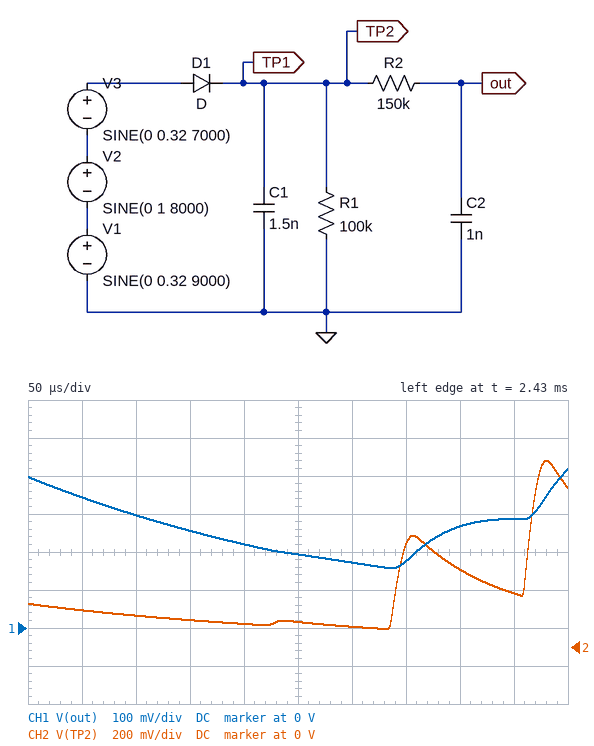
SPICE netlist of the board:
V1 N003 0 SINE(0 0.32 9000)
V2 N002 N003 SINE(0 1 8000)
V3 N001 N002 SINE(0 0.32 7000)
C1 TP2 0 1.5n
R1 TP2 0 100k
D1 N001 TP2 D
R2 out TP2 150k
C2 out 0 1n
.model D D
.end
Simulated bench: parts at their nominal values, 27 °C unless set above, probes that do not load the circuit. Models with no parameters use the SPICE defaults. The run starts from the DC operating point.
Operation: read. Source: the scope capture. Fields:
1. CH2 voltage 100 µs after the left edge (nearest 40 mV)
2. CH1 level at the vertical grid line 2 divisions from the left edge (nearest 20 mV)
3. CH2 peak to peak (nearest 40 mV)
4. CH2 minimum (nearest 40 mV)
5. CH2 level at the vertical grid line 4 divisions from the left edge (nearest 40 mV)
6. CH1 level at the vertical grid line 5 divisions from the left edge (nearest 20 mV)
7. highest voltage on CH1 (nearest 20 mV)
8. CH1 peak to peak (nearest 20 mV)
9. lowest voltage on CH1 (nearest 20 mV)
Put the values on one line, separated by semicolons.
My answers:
160 mV; 300 mV; 880 mV; 80 mV; 120 mV; 200 mV; 420 mV; 260 mV; 160 mV
